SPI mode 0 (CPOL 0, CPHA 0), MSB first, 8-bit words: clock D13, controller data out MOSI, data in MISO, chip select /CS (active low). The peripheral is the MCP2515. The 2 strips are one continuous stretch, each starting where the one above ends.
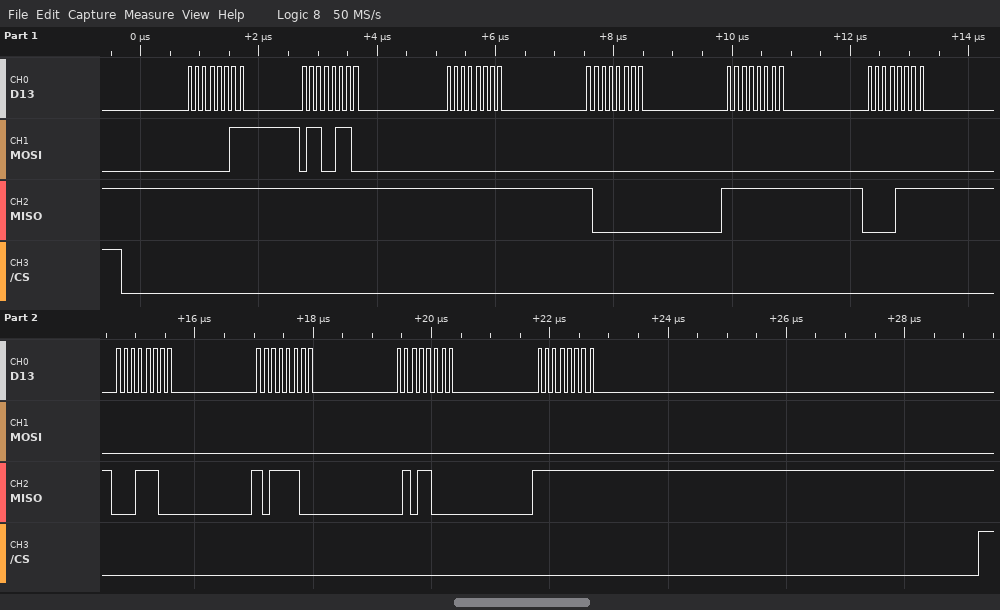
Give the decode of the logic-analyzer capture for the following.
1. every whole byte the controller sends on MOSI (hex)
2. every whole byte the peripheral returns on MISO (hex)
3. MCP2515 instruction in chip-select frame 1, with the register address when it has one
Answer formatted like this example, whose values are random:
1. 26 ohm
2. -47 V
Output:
1. 03 66 00 00 00 00 00 00 00 00
2. FF FF FF 80 FF 0F 1C BC 58 FF
3. READ 0x66
